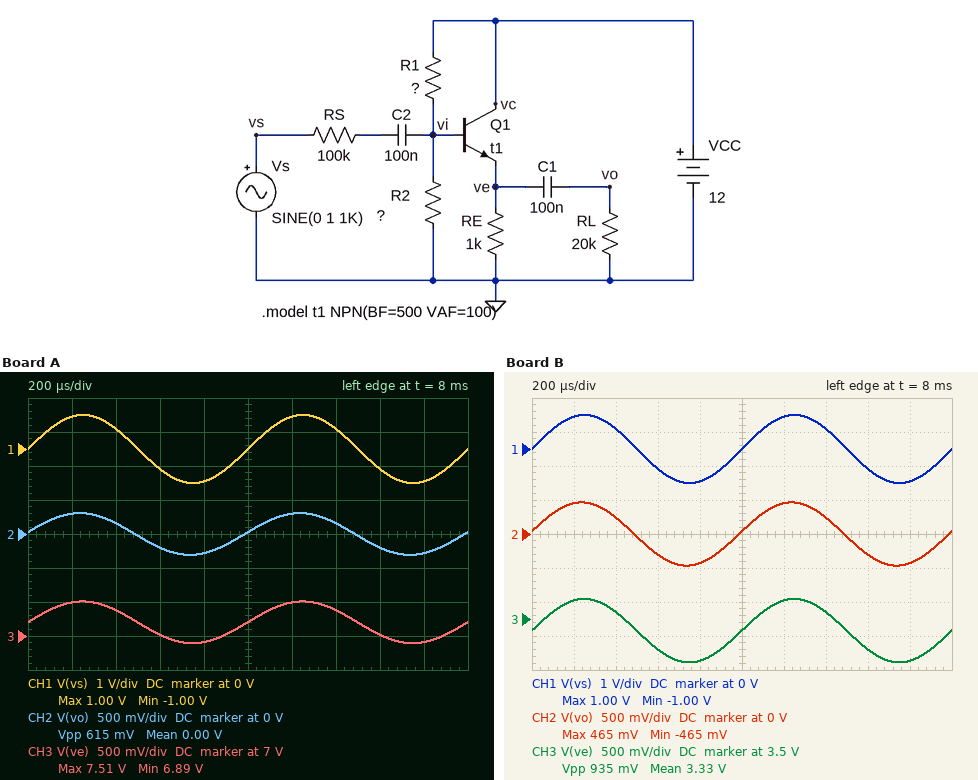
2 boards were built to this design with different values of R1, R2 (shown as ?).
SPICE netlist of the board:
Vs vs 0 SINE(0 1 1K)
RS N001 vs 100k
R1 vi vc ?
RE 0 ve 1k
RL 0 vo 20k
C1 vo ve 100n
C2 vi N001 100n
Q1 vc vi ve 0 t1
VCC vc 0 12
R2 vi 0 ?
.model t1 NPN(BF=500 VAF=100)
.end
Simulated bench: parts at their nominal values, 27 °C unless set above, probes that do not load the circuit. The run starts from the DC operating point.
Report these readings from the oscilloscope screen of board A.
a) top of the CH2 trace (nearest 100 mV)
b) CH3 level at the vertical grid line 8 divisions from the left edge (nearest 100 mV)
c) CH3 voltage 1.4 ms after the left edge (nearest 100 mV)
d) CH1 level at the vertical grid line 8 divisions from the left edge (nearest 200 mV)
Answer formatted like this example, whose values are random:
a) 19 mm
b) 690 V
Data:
a) 300 mV
b) 7.0 V
c) 7.4 V
d) -600 mV
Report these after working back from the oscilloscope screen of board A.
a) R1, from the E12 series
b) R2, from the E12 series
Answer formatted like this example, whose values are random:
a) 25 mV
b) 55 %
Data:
a) 68 kΩ
b) 180 kΩ
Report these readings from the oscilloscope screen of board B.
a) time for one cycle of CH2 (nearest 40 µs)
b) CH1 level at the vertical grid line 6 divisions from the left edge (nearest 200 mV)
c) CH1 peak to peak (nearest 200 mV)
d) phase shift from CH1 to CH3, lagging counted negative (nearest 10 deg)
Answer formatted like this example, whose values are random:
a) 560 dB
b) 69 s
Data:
a) 1.00 ms
b) 1.0 V
c) 2.0 V
d) 0 deg
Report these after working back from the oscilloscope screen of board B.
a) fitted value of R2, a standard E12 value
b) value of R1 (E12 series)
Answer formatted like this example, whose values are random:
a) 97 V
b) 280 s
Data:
a) 180 kΩ
b) 270 kΩ
